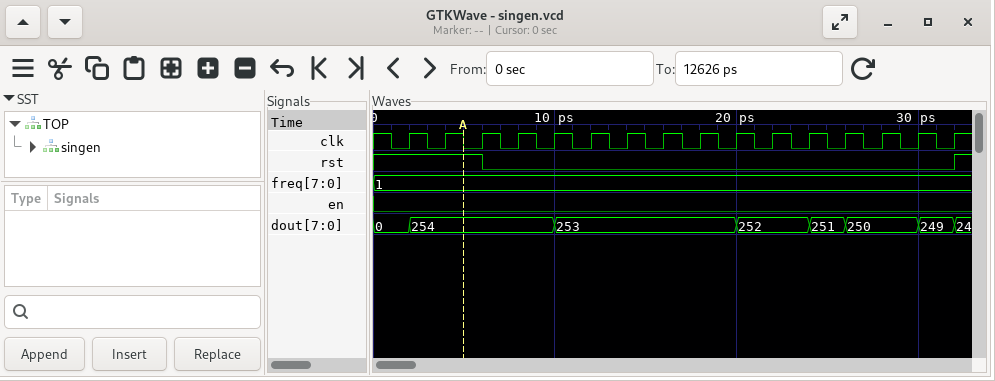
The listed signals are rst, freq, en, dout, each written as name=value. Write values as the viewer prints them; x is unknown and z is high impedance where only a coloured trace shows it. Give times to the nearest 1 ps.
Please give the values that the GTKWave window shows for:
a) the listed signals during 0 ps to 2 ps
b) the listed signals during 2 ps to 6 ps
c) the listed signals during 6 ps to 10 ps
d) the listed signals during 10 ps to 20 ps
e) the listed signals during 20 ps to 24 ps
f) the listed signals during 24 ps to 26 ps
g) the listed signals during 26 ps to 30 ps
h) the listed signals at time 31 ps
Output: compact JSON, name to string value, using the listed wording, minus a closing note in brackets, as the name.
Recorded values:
{"the listed signals during 0 ps to 2 ps": "rst=1, freq=1, en=0, dout=0", "the listed signals during 2 ps to 6 ps": "rst=1, freq=1, en=0, dout=254", "the listed signals during 6 ps to 10 ps": "rst=0, freq=1, en=0, dout=254", "the listed signals during 10 ps to 20 ps": "rst=0, freq=1, en=0, dout=253", "the listed signals during 20 ps to 24 ps": "rst=0, freq=1, en=0, dout=252", "the listed signals during 24 ps to 26 ps": "rst=0, freq=1, en=0, dout=251", "the listed signals during 26 ps to 30 ps": "rst=0, freq=1, en=0, dout=250", "the listed signals at time 31 ps": "rst=0, freq=1, en=0, dout=249"}
